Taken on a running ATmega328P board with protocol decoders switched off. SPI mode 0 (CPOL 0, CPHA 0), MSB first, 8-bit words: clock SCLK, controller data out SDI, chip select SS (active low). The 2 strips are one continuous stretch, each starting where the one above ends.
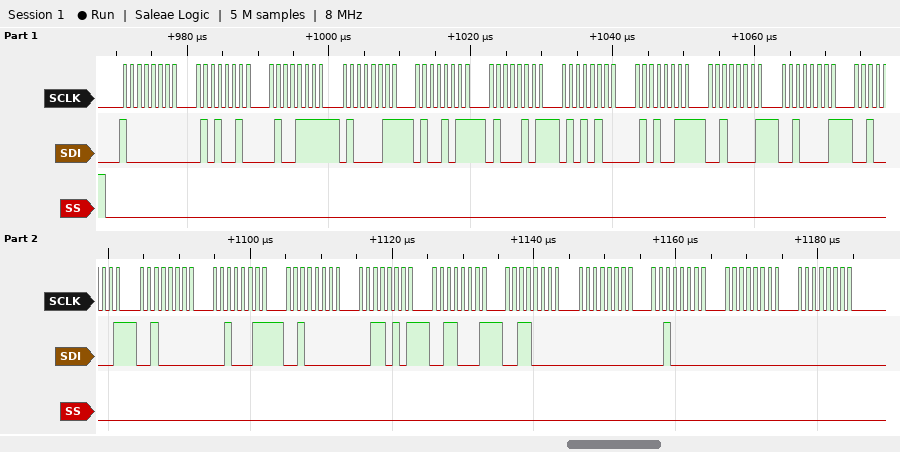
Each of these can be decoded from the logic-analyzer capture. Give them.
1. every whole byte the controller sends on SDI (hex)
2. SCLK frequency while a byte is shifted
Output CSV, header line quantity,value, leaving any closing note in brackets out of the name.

quantity,value
every whole byte the controller sends on SDI,80 52 4F 43 4B 45 54 53 21 21 21 20 23 20 35 31 30 00 20 00 00
SCLK frequency while a byte is shifted,1 MHz
